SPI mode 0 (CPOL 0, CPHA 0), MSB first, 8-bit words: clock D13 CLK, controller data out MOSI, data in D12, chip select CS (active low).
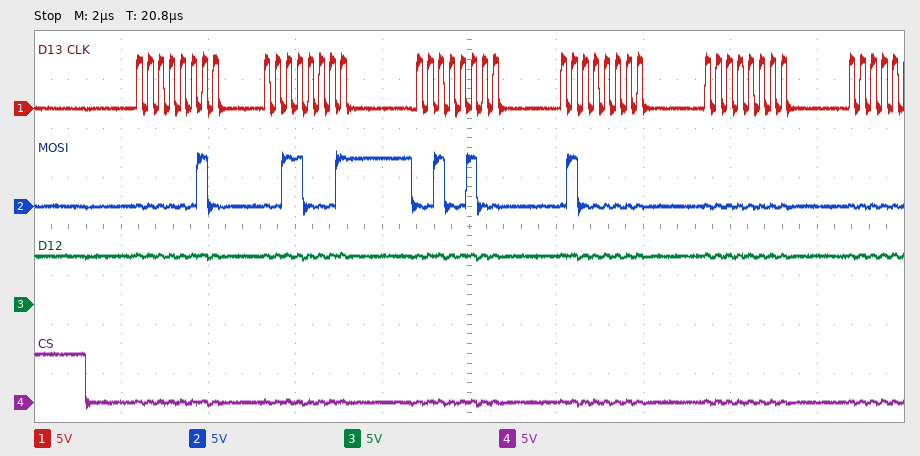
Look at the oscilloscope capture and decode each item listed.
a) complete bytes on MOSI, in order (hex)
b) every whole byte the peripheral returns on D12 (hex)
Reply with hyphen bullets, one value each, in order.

- 0x02 0x31 0x24 0x40 0x00
- 0xFF 0xFF 0xFF 0xFF 0xFF
